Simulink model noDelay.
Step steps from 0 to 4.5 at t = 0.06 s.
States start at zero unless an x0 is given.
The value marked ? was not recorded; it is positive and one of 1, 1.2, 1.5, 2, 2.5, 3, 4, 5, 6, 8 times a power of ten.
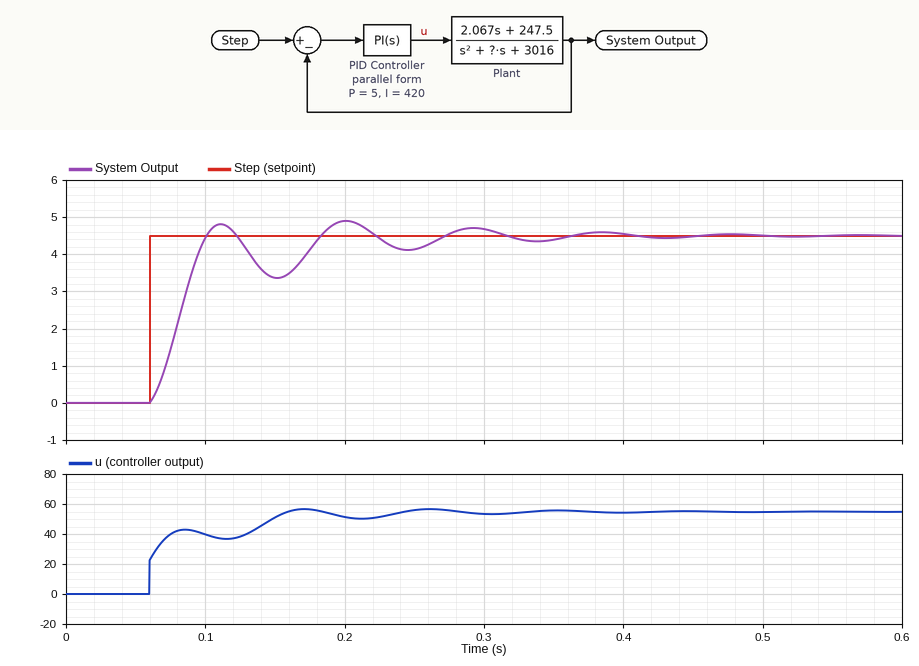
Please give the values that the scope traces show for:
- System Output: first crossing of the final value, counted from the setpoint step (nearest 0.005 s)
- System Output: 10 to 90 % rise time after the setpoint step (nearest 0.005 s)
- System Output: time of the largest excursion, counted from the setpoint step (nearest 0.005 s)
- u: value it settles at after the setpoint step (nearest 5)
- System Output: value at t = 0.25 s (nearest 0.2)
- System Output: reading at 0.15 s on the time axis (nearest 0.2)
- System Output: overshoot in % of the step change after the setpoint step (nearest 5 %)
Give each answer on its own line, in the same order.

0.040 s
0.030 s
0.140 s
55
4.2
3.4
10 %
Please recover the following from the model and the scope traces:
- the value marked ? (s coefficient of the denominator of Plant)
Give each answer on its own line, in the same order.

30
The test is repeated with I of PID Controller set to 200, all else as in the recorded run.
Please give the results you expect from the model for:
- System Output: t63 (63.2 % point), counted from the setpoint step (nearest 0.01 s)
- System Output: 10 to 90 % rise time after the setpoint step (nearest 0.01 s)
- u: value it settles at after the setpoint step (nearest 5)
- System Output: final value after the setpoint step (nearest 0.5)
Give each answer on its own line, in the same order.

0.03 s
0.13 s
55
4.5
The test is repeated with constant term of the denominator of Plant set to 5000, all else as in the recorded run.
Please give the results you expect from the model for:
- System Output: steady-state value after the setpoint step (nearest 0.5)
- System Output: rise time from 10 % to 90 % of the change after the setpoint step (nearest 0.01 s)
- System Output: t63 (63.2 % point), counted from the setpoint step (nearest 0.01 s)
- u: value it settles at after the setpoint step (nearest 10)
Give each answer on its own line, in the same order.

4.5
0.10 s
0.03 s
90
